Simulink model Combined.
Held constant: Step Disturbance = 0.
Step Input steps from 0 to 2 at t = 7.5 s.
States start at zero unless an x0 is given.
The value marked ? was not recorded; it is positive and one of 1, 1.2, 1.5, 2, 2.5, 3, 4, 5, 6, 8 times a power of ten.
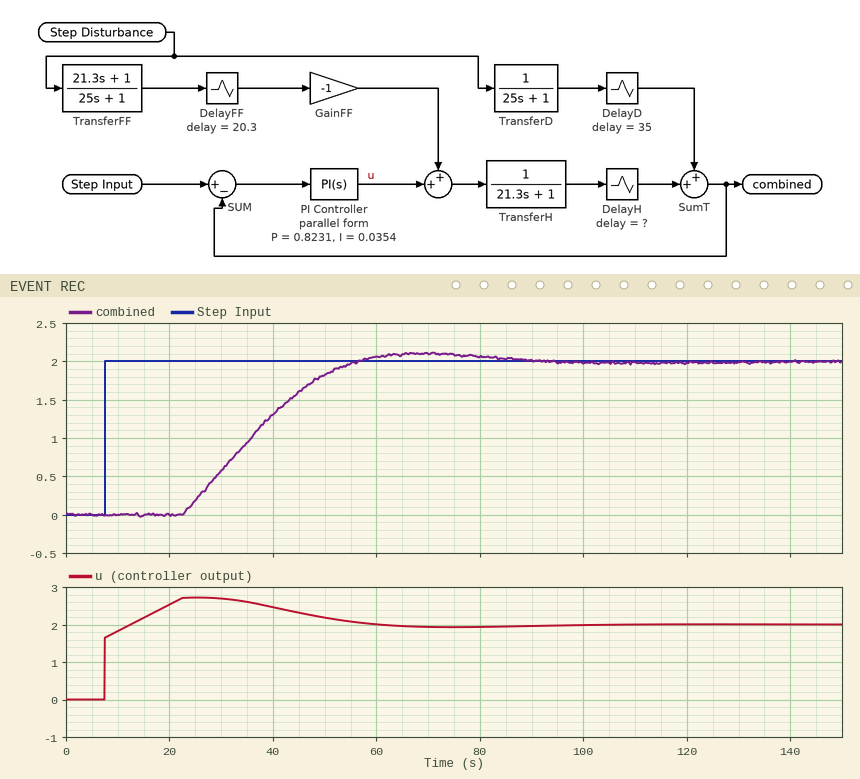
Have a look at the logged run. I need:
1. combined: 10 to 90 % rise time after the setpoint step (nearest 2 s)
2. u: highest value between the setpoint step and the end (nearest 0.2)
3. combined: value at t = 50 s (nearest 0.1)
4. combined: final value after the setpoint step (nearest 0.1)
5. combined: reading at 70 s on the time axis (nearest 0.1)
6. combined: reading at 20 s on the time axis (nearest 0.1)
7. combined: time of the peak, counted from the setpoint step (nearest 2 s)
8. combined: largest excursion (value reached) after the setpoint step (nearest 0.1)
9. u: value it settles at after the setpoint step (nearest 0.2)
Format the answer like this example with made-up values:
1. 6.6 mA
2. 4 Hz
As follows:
1. 24 s
2. 2.8
3. 1.8
4. 2.0
5. 2.1
6. 0.0
7. 62 s
8. 2.1
9. 2.0
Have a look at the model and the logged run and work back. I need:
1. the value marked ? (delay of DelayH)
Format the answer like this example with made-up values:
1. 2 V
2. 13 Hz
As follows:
1. 15
